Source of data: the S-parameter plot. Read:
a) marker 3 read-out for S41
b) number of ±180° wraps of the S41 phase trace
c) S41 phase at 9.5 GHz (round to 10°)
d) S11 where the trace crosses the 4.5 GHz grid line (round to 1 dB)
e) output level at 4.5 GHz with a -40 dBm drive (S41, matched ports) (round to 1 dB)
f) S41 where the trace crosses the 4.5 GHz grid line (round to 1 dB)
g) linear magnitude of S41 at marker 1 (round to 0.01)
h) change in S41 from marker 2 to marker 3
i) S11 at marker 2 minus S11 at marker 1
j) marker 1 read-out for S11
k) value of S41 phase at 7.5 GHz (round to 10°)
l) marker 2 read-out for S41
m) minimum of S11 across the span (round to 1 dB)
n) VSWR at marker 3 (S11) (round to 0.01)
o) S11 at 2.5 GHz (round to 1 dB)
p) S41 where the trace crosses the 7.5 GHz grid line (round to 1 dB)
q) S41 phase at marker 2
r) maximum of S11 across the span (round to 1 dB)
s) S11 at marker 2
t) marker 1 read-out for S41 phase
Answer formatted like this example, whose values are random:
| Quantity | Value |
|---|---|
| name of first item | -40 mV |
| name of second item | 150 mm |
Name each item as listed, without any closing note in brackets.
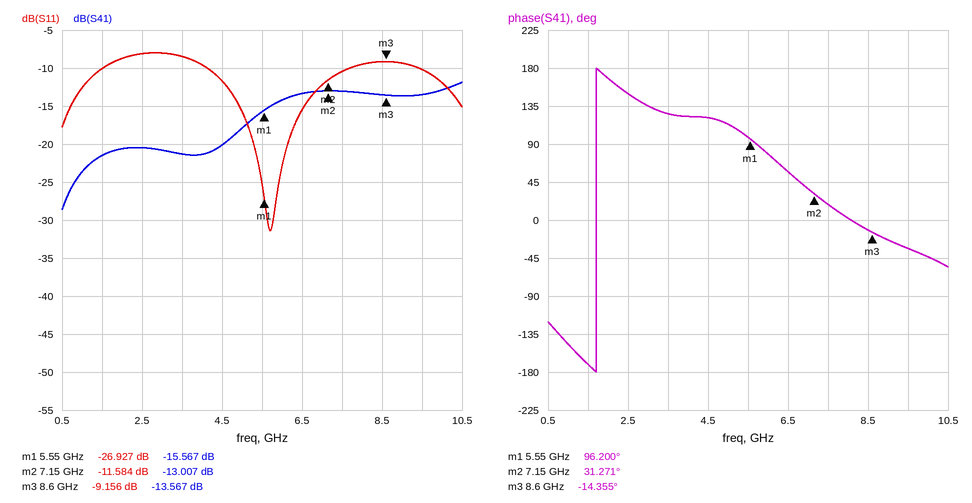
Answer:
| Quantity | Value |
|---|---|
| marker 3 read-out for S41 | -13.567 dB |
| number of ±180° wraps of the S41 phase trace | 1 |
| S41 phase at 9.5 GHz | -30° |
| S11 where the trace crosses the 4.5 GHz grid line | -12 dB |
| output level at 4.5 GHz with a -40 dBm drive (S41, matched ports) | -60 dBm |
| S41 where the trace crosses the 4.5 GHz grid line | -20 dB |
| linear magnitude of S41 at marker 1 | 0.17 |
| change in S41 from marker 2 to marker 3 | -0.560 dB |
| S11 at marker 2 minus S11 at marker 1 | 15.343 dB |
| marker 1 read-out for S11 | -26.927 dB |
| value of S41 phase at 7.5 GHz | 20° |
| marker 2 read-out for S41 | -13.007 dB |
| minimum of S11 across the span | -31 dB |
| VSWR at marker 3 (S11) | 2.07 |
| S11 at 2.5 GHz | -8 dB |
| S41 where the trace crosses the 7.5 GHz grid line | -13 dB |
| S41 phase at marker 2 | 31.271° |
| maximum of S11 across the span | -8 dB |
| S11 at marker 2 | -11.584 dB |
| marker 1 read-out for S41 phase | 96.200° |
